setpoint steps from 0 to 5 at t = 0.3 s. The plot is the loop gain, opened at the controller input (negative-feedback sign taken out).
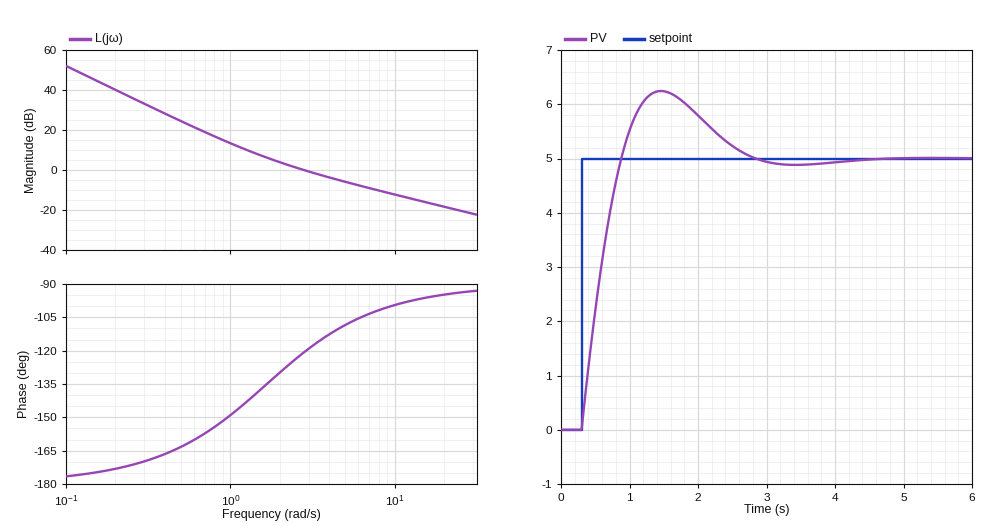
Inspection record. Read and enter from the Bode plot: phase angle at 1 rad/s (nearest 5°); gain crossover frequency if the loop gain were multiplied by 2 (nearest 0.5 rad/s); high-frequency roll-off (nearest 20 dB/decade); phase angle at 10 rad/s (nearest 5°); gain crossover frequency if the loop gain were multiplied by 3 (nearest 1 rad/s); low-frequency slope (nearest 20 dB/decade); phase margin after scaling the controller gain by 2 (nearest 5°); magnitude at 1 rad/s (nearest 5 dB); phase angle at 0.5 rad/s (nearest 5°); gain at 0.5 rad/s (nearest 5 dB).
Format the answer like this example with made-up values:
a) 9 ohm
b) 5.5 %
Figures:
a) -150°
b) 5.0 rad/s
c) -20 dB/decade
d) -100°
e) 7 rad/s
f) -40 dB/decade
g) 70°
h) 15 dB
i) -165°
j) 25 dB
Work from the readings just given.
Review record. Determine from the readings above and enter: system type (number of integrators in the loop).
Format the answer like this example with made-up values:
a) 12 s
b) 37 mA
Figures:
a) 2
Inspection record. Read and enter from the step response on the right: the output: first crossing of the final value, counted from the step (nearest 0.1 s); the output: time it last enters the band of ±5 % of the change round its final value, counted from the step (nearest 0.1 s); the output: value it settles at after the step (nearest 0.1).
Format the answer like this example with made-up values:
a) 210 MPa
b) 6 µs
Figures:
a) 0.6 s
b) 2.2 s
c) 5.0
